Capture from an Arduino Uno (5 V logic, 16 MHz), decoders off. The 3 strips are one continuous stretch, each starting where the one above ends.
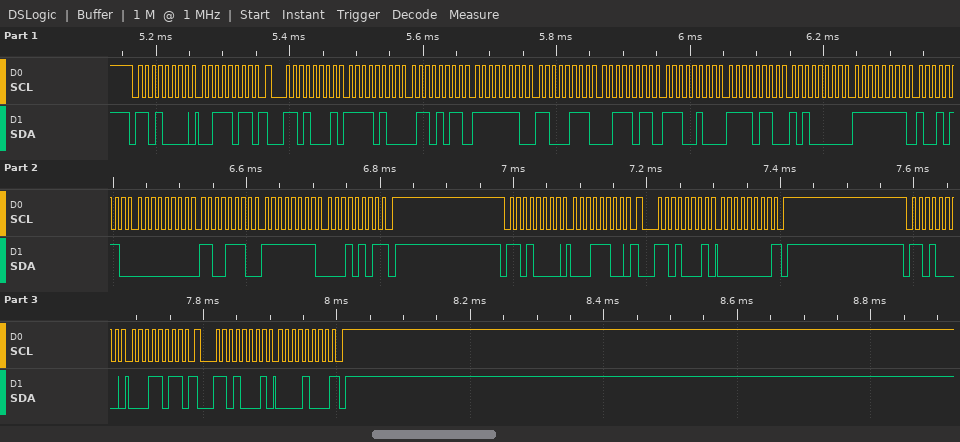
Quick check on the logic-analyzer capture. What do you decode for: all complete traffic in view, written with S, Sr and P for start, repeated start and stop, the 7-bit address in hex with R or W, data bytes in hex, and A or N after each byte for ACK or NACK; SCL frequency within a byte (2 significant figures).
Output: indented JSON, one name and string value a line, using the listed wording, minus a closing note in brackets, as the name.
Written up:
{
  "all complete traffic in view, written with S, Sr and P for start, repeated start and stop, the 7-bit address in hex with R or W, data bytes in hex, and A or N after each byte for ACK or NACK": "S 68W A 3B A Sr 68R A F4 A 6B A FE A C7 A 3B A E4 A F6 A A0 A FF A 96 A 00 A CE A FF A 15 N P S 68W A 1C A Sr 68R A 00 N P S 68W A 1B A Sr 68R A 08 N P",
  "SCL frequency within a byte": "100 kHz"
}
